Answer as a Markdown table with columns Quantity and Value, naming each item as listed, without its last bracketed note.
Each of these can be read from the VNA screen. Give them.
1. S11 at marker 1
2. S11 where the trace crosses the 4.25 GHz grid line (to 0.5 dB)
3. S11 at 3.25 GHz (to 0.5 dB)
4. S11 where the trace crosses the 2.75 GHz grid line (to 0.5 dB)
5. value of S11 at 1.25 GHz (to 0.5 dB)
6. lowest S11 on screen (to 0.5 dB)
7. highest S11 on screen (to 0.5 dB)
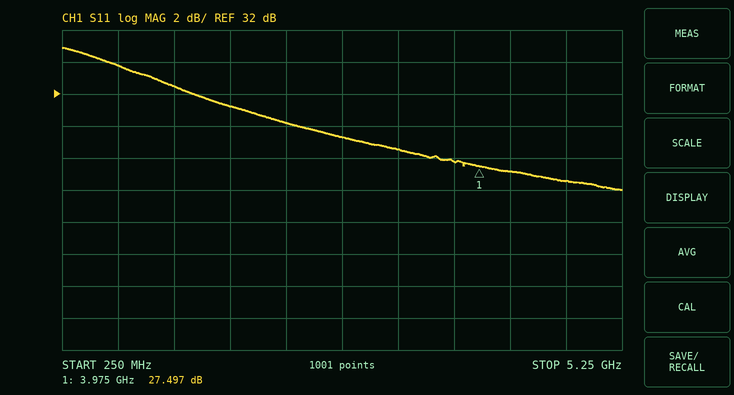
| Quantity | Value |
|---|---|
| S11 at marker 1 | 27.497 dB |
| S11 where the trace crosses the 4.25 GHz grid line | 27.0 dB |
| S11 at 3.25 GHz | 28.5 dB |
| S11 where the trace crosses the 2.75 GHz grid line | 29.5 dB |
| value of S11 at 1.25 GHz | 32.5 dB |
| lowest S11 on screen | 26.0 dB |
| highest S11 on screen | 35.0 dB |
